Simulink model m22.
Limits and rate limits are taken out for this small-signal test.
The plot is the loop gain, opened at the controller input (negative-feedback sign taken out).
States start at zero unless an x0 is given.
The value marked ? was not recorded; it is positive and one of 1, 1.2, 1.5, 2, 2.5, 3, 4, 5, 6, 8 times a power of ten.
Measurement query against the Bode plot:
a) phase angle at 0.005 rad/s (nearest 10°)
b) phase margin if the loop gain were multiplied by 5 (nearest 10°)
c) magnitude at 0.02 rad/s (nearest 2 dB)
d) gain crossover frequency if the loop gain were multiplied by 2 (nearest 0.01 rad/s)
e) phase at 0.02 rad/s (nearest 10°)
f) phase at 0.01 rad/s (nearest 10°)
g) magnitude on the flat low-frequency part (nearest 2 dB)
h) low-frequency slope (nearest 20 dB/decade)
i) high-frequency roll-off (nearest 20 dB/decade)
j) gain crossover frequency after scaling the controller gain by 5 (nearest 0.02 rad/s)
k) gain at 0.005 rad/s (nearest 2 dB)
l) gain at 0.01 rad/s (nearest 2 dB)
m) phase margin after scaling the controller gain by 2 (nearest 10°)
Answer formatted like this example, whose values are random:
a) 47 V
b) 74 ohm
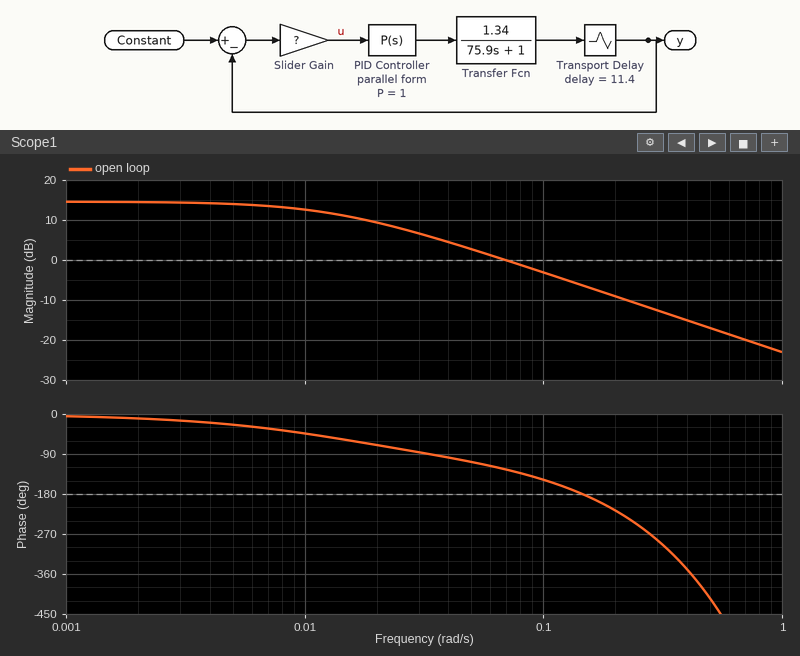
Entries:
a) -20°
b) -140°
c) 10 dB
d) 0.14 rad/s
e) -70°
f) -40°
g) 14 dB
h) 0 dB/decade
i) -20 dB/decade
j) 0.36 rad/s
k) 14 dB
l) 12 dB
m) 0°
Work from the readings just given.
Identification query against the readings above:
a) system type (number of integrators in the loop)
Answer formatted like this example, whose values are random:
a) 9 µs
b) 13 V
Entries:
a) 0
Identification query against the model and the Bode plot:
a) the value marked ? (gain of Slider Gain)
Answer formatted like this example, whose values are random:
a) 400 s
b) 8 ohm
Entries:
a) 4
